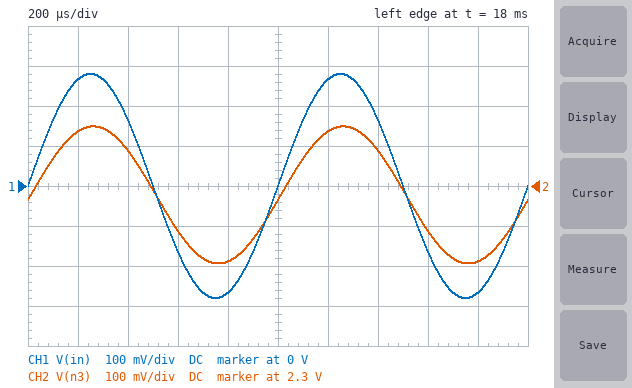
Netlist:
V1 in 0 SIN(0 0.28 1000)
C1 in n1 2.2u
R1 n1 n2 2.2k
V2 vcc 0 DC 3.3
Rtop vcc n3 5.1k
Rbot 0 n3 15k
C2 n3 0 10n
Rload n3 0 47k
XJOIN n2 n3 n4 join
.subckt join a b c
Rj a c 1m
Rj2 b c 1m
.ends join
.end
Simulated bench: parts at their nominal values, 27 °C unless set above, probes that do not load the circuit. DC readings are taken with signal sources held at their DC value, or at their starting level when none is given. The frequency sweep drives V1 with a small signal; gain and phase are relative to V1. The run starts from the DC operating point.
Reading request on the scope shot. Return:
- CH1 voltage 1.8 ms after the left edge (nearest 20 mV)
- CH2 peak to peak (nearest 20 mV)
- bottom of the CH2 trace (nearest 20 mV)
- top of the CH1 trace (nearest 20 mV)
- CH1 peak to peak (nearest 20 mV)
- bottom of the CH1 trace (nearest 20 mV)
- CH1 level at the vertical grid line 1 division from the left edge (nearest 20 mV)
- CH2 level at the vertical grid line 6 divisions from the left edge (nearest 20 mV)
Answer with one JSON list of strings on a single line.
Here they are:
["-260 mV", "340 mV", "2.10 V", "280 mV", "560 mV", "-280 mV", "260 mV", "2.44 V"]
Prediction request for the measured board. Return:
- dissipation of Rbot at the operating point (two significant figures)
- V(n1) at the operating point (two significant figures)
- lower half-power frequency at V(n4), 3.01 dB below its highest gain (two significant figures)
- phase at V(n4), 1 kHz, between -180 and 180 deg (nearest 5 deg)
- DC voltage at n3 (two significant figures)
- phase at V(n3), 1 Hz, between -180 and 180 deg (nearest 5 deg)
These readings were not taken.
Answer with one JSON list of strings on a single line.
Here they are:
["350 µW", "2.3 V", "13 Hz", "-5 deg", "2.3 V", "85 deg"]
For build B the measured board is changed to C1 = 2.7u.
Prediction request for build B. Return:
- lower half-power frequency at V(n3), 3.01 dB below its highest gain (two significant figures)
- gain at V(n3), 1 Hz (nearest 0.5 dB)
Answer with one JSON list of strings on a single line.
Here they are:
["10 Hz", "-24.5 dB"]
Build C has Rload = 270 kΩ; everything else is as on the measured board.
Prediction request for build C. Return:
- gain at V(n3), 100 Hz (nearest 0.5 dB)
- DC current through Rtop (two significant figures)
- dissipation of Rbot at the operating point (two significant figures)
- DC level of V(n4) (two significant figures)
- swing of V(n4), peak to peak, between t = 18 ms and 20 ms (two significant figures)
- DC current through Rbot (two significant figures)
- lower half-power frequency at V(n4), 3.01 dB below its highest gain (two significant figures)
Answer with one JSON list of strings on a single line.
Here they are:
["-4.0 dB", "170 µA", "390 µW", "2.4 V", "350 mV", "160 µA", "12 Hz"]
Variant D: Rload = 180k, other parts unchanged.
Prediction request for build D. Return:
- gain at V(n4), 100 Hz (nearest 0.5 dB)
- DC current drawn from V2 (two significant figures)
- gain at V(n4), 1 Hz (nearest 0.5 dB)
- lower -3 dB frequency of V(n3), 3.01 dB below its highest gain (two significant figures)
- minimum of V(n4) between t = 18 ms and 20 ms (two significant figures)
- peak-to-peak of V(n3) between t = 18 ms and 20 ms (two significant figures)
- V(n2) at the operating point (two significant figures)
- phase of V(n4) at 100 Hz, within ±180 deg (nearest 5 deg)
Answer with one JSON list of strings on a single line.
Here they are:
["-4.0 dB", "170 µA", "-26.0 dB", "12 Hz", "2.2 V", "350 mV", "2.4 V", "5 deg"]
